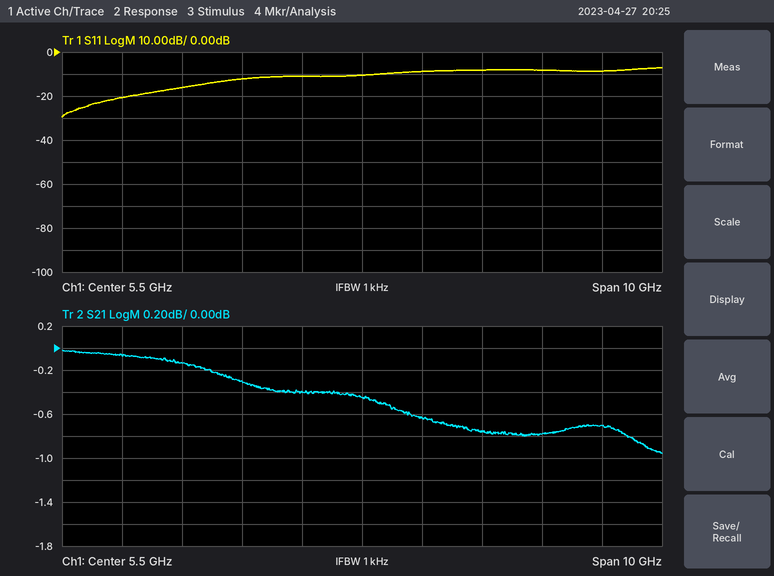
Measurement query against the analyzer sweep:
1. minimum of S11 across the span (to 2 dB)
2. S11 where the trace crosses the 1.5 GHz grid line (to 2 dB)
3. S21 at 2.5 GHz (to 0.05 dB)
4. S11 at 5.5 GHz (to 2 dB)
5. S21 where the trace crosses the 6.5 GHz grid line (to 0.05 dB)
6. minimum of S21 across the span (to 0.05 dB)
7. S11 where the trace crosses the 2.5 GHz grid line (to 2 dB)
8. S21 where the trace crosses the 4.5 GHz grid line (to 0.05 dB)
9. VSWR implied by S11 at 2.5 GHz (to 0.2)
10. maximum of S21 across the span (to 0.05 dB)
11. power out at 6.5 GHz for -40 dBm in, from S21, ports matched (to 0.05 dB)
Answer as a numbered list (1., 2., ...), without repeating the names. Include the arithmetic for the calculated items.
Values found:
1. -30 dB
2. -20 dB
3. -0.15 dB
4. -10 dB
5. -0.65 dB
6. -0.95 dB
7. -16 dB
8. -0.40 dB
9. |Γ| = 10^(-16/20) = 0.1585; VSWR = (1 + 0.1585)/(1 − 0.1585) ≈ 1.4
10. 0.00 dB
11. -40 dBm + (-0.65 dB) = -40.65 dBm
